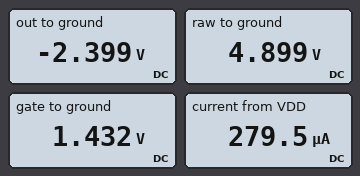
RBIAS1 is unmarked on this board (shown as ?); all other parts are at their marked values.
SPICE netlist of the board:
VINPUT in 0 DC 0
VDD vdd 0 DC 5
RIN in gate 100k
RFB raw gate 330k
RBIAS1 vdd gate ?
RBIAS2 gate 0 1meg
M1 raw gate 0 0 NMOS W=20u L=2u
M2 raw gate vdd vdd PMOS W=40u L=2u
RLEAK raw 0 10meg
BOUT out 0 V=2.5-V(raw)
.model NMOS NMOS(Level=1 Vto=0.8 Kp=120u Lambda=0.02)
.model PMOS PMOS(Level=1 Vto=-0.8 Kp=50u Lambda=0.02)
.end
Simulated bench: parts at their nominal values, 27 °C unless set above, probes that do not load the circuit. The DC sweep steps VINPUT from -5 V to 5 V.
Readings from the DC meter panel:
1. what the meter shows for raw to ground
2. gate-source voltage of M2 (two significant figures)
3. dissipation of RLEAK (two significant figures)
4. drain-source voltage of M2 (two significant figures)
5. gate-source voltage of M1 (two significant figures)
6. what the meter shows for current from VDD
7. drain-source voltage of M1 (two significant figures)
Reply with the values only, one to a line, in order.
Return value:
4.899 V
-3.6 V
2.4 µW
-100 mV
1.4 V
279.5 µA
4.9 V
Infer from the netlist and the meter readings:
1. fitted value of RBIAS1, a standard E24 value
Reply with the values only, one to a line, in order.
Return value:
680 kΩ
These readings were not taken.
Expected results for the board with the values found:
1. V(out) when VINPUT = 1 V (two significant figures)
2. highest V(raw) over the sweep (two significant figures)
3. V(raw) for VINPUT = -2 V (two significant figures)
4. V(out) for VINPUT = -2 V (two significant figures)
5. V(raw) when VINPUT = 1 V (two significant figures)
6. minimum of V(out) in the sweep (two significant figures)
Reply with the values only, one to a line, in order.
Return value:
-2.0 V
5.0 V
5.0 V
-2.5 V
4.5 V
-2.5 V
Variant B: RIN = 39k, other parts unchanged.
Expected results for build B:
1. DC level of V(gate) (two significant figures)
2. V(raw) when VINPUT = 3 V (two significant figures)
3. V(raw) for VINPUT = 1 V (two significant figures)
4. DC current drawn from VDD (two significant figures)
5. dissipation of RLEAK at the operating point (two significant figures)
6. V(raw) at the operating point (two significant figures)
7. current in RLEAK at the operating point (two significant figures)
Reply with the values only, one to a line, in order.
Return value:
720 mV
560 mV
4.9 V
20 µA
2.5 µW
5.0 V
500 nA
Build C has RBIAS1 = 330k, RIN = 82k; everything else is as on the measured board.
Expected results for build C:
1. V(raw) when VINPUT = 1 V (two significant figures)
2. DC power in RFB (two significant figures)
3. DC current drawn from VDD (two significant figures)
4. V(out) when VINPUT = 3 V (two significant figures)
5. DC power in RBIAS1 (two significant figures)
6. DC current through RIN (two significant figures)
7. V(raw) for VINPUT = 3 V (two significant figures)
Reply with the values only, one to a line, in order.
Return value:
4.4 V
33 µW
390 µA
2.0 V
36 µW
19 µA
540 mV
